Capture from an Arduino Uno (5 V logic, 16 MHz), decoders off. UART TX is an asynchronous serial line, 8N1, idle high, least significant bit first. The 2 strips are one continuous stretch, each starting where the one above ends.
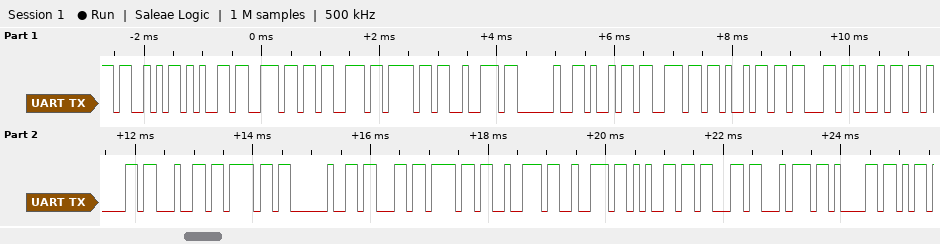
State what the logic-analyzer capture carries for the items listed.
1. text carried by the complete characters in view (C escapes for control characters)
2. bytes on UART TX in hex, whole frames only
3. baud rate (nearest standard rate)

"Sensor iniciado correcta"
53 65 6E 73 6F 72 20 69 6E 69 63 69 61 64 6F 20 63 6F 72 72 65 63 74 61
9600 baud
